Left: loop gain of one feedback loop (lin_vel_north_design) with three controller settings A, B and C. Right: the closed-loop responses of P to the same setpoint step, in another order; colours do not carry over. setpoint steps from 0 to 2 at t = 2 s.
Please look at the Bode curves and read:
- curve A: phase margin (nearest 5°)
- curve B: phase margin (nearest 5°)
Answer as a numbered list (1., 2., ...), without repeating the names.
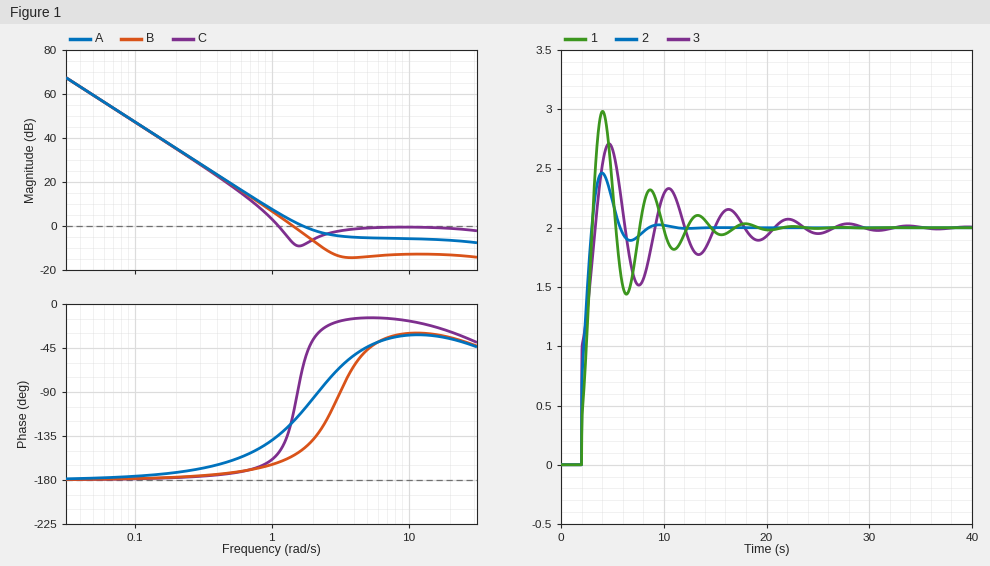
1. 70°
2. 25°
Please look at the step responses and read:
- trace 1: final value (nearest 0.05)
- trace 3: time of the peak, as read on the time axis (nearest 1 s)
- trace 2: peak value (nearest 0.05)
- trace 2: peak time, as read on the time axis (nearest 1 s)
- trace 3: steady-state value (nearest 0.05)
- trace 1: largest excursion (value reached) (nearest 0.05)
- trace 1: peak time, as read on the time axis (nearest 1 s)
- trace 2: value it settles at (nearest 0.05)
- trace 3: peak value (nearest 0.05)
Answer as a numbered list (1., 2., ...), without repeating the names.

1. 2.00
2. 5 s
3. 2.45
4. 4 s
5. 2.00
6. 3.00
7. 4 s
8. 2.00
9. 2.70
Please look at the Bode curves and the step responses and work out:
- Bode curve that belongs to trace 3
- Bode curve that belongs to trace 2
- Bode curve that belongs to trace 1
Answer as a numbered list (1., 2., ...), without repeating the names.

1. C
2. A
3. B
